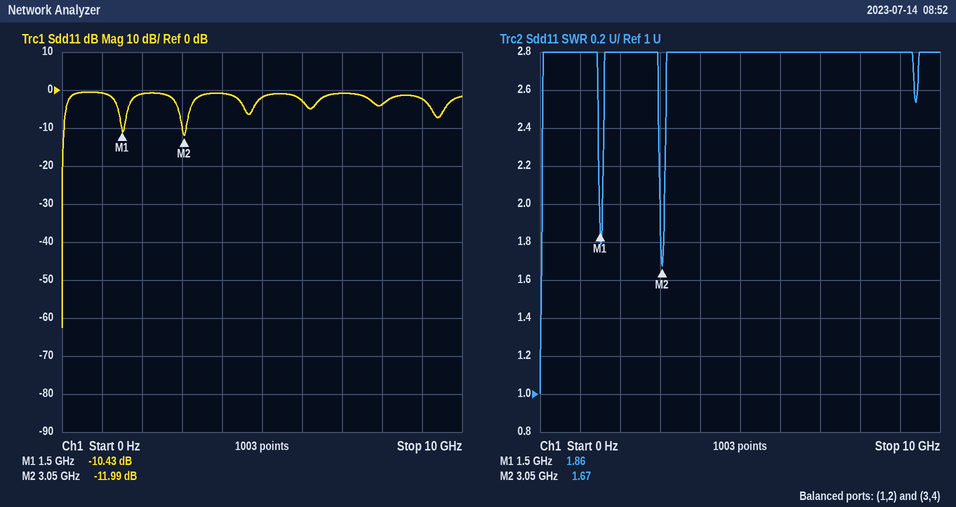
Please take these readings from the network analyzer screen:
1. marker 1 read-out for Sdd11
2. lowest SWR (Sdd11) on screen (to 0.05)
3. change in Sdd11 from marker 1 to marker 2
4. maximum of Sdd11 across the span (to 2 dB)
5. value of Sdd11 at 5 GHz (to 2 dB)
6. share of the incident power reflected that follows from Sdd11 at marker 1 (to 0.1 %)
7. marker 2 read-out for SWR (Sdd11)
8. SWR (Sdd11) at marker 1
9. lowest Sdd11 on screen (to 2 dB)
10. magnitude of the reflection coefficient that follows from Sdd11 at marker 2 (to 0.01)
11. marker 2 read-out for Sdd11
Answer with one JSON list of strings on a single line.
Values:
["-10.43 dB", "1.00", "-1.56 dB", "0 dB", "-2 dB", "9.1 %", "1.67", "1.86", "-62 dB", "0.25", "-11.99 dB"]
